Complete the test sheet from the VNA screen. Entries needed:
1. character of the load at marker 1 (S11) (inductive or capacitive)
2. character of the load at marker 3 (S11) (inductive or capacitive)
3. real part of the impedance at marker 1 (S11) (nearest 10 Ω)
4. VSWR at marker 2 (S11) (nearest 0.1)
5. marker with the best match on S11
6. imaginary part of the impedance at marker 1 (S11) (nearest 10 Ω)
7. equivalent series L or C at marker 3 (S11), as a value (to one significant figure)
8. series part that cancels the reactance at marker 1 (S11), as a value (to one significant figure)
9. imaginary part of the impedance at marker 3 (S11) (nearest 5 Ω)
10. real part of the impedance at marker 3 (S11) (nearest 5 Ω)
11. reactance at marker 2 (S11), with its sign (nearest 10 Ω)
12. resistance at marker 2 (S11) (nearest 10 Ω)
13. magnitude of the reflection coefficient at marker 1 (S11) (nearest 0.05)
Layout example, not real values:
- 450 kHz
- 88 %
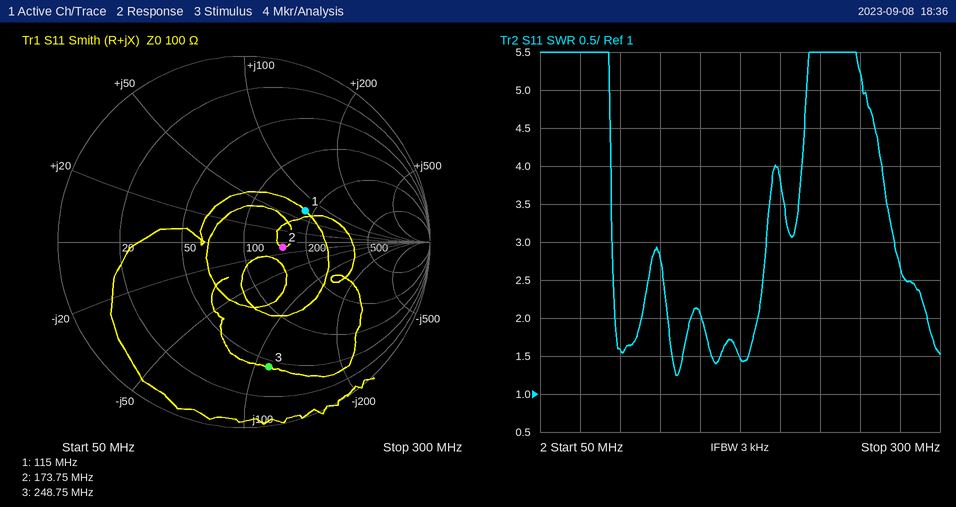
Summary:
- inductive
- capacitive
- 180 Ω
- 1.5
- marker 2
- +70 Ω
- 6 pF
- 20 pF
- -110 Ω
- 45 Ω
- -10 Ω
- 150 Ω
- 0.35
